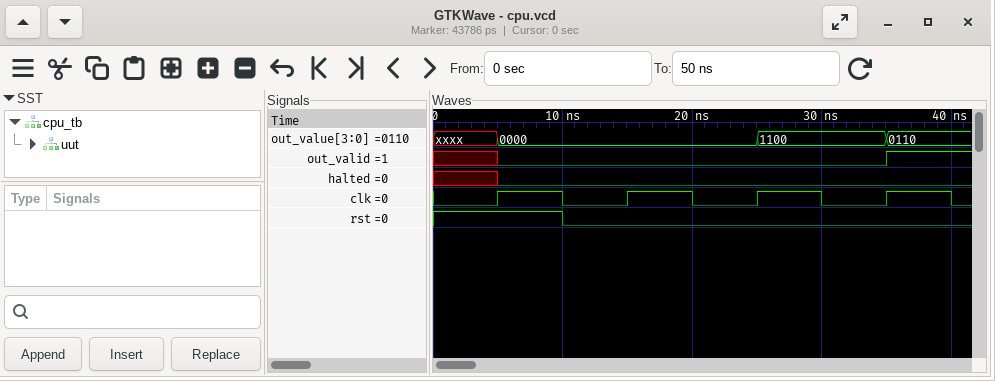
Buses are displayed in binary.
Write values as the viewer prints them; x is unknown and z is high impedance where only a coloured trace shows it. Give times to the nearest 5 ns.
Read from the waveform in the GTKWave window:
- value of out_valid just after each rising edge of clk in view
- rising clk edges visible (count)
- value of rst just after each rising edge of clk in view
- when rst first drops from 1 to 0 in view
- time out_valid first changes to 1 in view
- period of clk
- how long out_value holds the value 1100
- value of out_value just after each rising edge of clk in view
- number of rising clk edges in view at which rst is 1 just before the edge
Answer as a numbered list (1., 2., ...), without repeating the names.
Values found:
1. 0 0 0 1
2. 4
3. 1 0 0 0
4. 10 ns
5. 35 ns
6. 10 ns
7. 10 ns
8. 0000, 0000, 1100, 0110
9. 1
